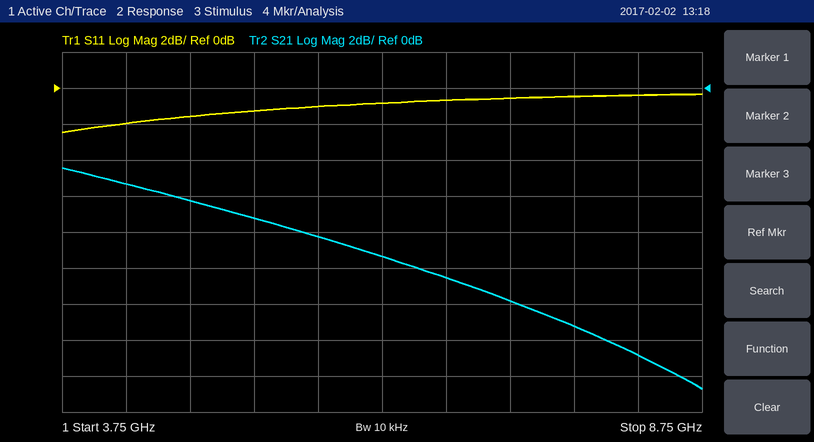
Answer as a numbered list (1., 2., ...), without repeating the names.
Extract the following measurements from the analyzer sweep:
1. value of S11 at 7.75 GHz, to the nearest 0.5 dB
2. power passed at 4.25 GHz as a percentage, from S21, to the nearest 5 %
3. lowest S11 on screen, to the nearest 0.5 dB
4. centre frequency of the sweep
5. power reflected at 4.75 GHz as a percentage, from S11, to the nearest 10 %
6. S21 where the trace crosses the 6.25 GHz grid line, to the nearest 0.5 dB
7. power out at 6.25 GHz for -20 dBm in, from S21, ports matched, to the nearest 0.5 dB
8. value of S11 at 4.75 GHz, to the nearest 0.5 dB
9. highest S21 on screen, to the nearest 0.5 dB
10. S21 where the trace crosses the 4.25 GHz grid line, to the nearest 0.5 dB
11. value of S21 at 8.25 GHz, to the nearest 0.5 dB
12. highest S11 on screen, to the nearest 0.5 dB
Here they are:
1. -0.5 dB
2. 30 %
3. -2.5 dB
4. 6.25 GHz
5. 70 %
6. -9.5 dB
7. -29.5 dBm
8. -1.5 dB
9. -4.5 dB
10. -5.5 dB
11. -15.0 dB
12. -0.5 dB
